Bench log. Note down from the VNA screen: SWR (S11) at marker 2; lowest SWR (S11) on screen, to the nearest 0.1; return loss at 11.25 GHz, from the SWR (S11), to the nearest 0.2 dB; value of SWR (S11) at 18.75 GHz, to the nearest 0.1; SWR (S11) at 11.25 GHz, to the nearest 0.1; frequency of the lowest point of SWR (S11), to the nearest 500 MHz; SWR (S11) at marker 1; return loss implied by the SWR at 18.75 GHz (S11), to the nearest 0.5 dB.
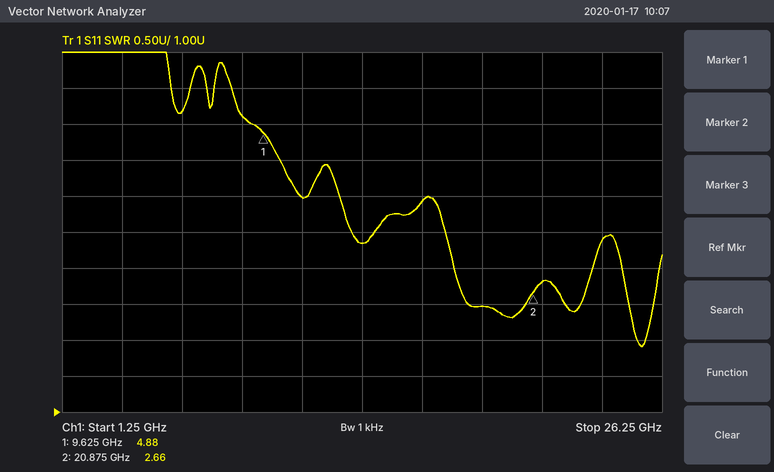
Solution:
2.66
1.9
4.4 dB
2.5
4.0
25.5 GHz
4.88
7.5 dB
